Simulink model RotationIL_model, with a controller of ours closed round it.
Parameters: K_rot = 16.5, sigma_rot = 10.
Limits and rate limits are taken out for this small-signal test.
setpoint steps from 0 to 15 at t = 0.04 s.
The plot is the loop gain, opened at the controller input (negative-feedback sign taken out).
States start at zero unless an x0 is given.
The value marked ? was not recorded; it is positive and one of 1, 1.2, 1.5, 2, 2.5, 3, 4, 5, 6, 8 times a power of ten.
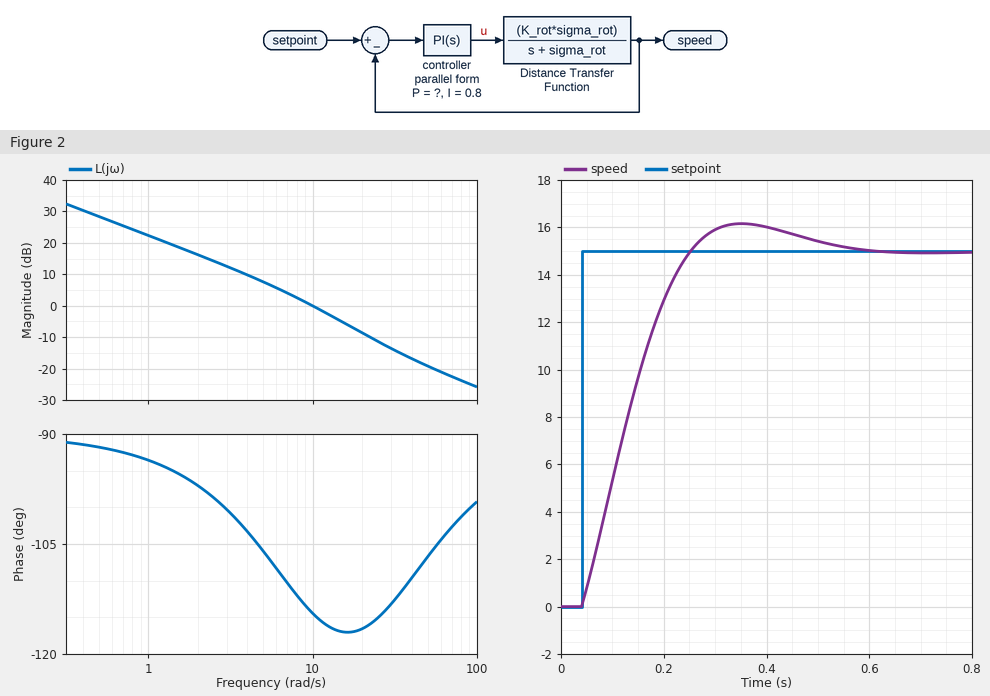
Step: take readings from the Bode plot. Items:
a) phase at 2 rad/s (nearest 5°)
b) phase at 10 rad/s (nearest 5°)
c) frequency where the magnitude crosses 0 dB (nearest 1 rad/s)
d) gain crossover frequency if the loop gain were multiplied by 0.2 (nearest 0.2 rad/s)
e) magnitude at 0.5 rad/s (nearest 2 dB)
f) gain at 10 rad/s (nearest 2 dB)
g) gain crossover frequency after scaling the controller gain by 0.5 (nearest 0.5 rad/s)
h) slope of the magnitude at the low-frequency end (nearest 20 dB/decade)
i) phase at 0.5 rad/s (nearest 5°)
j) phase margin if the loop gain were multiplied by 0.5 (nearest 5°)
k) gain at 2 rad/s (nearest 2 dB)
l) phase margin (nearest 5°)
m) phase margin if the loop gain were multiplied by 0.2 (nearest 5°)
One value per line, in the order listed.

-95°
-115°
10 rad/s
2.6 rad/s
28 dB
0 dB
6.0 rad/s
-20 dB/decade
-90°
70°
16 dB
65°
80°
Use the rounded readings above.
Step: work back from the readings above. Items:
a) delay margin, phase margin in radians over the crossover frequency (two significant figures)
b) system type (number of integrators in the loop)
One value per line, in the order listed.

0.11 s
1
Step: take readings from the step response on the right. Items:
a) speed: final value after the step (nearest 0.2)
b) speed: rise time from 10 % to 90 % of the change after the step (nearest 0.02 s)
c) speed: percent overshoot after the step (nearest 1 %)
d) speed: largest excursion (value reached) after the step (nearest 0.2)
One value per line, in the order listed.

15.0
0.16 s
8 %
16.2
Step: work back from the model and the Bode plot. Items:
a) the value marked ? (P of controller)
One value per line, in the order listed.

0.03
